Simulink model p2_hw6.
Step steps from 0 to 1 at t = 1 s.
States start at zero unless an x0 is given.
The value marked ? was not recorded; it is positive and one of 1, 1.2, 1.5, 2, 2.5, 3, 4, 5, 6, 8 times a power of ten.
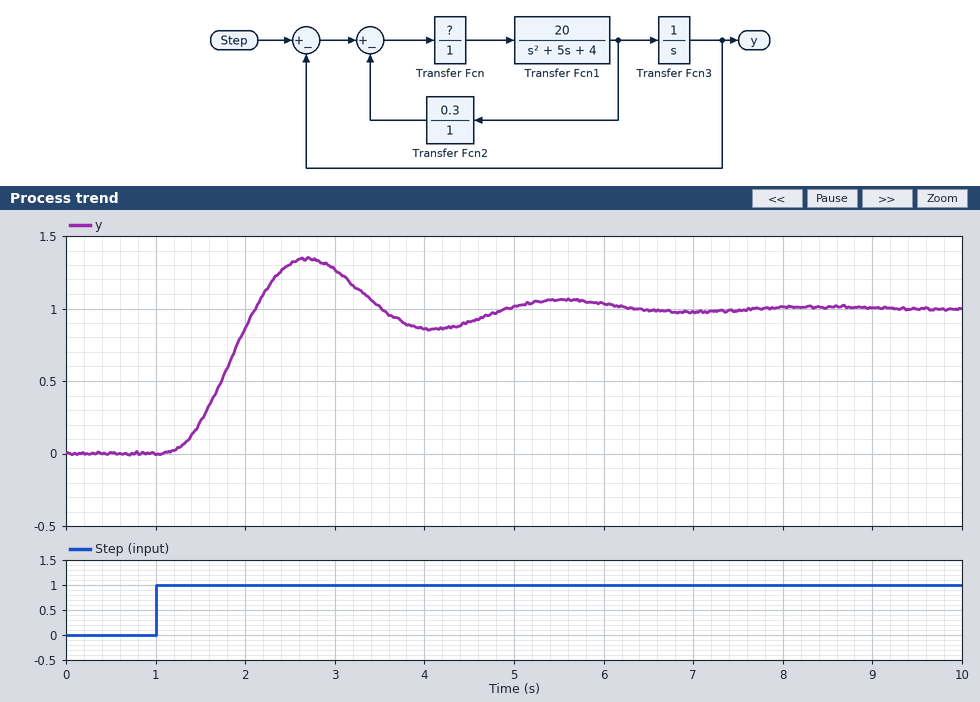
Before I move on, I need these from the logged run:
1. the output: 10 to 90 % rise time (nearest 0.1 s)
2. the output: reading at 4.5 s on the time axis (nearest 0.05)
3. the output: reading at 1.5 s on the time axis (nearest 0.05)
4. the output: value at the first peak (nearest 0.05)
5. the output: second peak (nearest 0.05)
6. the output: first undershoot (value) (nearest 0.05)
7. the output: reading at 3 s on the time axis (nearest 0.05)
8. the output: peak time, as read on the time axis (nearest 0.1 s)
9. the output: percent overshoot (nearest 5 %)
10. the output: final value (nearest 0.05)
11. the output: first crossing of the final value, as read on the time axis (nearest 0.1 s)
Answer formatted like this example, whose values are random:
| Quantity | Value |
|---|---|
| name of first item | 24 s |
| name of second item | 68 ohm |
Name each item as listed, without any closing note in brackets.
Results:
| Quantity | Value |
|---|---|
| the output: 10 to 90 % rise time | 0.7 s |
| the output: reading at 4.5 s on the time axis | 0.90 |
| the output: reading at 1.5 s on the time axis | 0.20 |
| the output: value at the first peak | 1.35 |
| the output: second peak | 1.05 |
| the output: first undershoot (value) | 0.85 |
| the output: reading at 3 s on the time axis | 1.25 |
| the output: peak time, as read on the time axis | 2.7 s |
| the output: percent overshoot | 35 % |
| the output: final value | 1.00 |
| the output: first crossing of the final value, as read on the time axis | 2.1 s |
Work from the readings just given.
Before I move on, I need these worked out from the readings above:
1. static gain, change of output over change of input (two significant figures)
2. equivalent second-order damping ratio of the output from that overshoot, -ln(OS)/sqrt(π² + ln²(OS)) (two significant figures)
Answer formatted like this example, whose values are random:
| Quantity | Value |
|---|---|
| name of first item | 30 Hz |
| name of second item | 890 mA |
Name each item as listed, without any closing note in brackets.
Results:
| Quantity | Value |
|---|---|
| static gain, change of output over change of input | 1.0 |
| equivalent second-order damping ratio of the output from that overshoot, -ln(OS)/sqrt(π² + ln²(OS)) | 0.32 |
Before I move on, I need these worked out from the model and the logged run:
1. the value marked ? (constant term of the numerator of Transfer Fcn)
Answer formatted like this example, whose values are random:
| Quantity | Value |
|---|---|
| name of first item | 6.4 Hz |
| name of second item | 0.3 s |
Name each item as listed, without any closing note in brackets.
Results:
| Quantity | Value |
|---|---|
| the value marked ? | 1 |
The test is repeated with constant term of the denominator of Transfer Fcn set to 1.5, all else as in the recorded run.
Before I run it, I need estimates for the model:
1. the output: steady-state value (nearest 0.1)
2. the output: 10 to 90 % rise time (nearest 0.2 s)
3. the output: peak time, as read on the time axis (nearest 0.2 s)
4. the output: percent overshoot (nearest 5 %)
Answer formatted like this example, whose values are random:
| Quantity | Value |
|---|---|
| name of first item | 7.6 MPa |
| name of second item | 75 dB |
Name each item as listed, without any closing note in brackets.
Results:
| Quantity | Value |
|---|---|
| the output: steady-state value | 1.0 |
| the output: 10 to 90 % rise time | 0.8 s |
| the output: peak time, as read on the time axis | 3.0 s |
| the output: percent overshoot | 30 % |
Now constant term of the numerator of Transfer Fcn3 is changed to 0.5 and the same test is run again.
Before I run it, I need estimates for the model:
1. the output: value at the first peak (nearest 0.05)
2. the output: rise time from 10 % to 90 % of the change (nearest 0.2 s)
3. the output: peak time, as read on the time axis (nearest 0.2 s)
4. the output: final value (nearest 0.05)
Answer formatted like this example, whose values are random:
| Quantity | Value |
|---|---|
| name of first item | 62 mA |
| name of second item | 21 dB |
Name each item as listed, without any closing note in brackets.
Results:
| Quantity | Value |
|---|---|
| the output: value at the first peak | 1.05 |
| the output: rise time from 10 % to 90 % of the change | 1.2 s |
| the output: peak time, as read on the time axis | 3.6 s |
| the output: final value | 1.00 |
